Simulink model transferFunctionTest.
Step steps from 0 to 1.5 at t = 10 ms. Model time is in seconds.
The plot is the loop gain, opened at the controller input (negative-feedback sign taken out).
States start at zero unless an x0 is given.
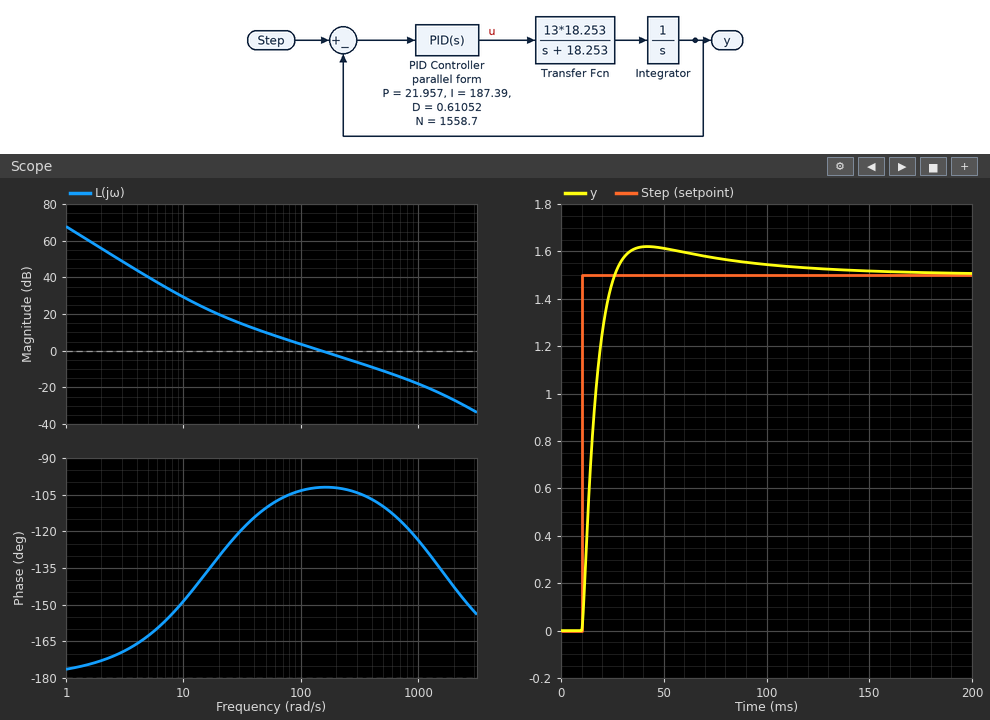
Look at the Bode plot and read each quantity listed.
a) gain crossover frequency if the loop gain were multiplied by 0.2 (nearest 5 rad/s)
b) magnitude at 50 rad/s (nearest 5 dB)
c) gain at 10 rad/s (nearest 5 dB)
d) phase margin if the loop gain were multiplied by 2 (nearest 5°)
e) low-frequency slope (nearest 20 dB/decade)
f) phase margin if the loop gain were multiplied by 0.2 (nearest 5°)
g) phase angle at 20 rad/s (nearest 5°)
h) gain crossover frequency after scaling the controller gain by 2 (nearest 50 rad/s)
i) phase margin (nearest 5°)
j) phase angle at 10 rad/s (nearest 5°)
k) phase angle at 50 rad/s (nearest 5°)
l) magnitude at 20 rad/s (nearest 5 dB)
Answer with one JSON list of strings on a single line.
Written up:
["35 rad/s", "10 dB", "30 dB", "75°", "-40 dB/decade", "60°", "-130°", "300 rad/s", "80°", "-150°", "-110°", "20 dB"]
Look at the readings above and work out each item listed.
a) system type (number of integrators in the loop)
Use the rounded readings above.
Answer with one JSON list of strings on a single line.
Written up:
["2"]
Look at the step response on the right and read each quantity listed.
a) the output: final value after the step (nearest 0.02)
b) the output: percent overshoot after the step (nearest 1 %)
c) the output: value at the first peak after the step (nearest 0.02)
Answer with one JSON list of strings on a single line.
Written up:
["1.50", "8 %", "1.62"]
